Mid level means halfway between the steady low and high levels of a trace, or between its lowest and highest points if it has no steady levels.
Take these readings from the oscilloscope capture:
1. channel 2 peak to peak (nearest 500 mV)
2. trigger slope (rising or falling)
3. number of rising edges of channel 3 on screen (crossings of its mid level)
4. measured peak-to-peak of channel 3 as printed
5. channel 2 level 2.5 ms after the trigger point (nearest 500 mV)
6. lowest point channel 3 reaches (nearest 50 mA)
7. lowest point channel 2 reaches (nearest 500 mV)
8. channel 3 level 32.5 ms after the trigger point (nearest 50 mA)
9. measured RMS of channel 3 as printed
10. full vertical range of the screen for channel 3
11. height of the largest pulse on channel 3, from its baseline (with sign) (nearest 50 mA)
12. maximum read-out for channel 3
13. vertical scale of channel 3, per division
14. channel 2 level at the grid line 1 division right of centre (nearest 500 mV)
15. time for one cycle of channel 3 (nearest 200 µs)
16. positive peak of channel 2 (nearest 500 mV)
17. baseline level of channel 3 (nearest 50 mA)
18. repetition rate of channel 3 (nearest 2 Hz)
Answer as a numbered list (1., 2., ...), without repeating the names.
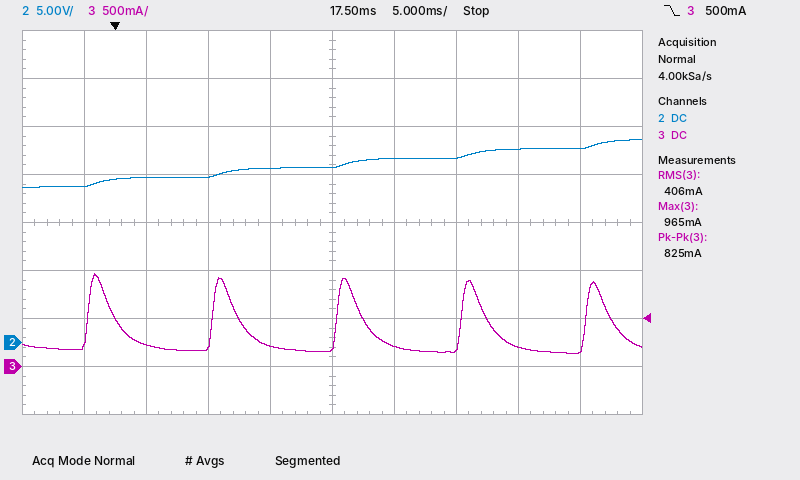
1. 5.0 V
2. falling
3. 5
4. 825 mA
5. 17.0 V
6. 150 mA
7. 16.0 V
8. 200 mA
9. 406 mA
10. 4 A
11. +800 mA
12. 965 mA
13. 500 mA
14. 19.0 V
15. 10.0 ms
16. 21.0 V
17. 200 mA
18. 100 Hz
